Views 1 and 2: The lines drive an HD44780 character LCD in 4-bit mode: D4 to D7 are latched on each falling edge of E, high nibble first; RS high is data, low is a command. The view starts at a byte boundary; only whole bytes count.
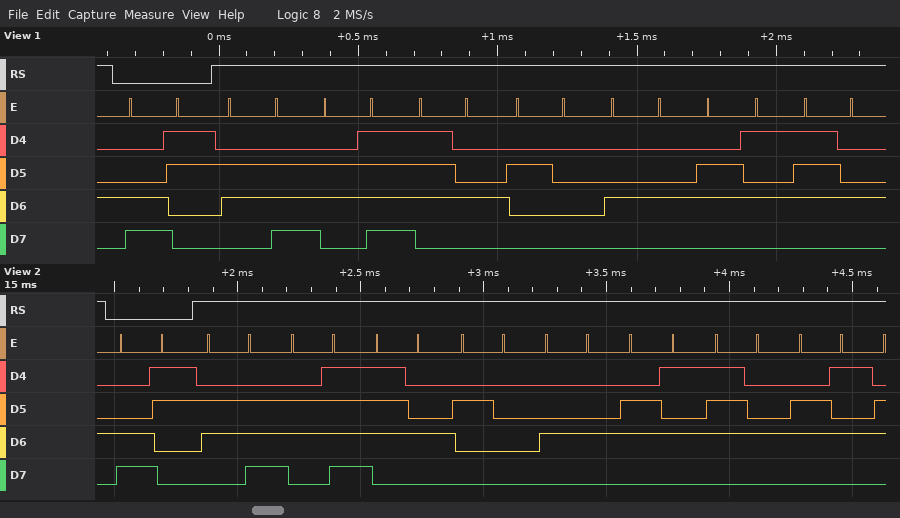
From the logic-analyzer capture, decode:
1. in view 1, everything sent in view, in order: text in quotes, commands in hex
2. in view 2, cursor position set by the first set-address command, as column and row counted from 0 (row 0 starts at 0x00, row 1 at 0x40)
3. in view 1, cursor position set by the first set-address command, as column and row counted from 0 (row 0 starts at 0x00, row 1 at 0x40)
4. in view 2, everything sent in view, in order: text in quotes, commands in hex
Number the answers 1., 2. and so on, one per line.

1. 0xC3 "not Det"
2. column 3, row 1
3. column 3, row 1
4. 0xC3 "not Dete"
